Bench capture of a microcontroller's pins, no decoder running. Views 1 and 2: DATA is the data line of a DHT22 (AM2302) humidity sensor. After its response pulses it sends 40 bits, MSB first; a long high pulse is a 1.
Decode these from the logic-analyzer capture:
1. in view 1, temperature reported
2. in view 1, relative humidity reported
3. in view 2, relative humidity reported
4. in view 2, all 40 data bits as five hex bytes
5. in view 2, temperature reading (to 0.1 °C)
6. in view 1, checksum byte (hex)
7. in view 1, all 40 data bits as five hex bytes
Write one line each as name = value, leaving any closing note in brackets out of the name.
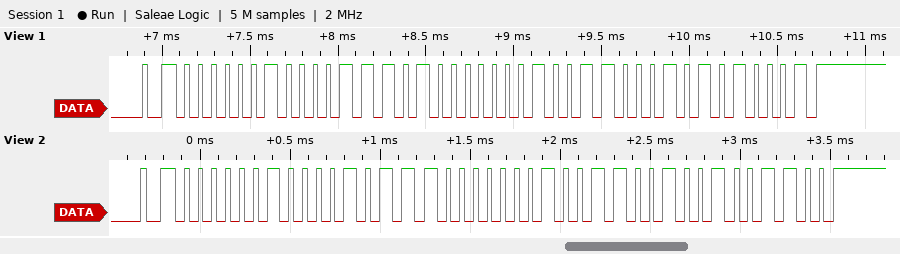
in view 1, temperature reported = 30.5 °C
in view 1, relative humidity reported = 54.1 %
in view 2, relative humidity reported = 53.5 %
in view 2, all 40 data bits as five hex bytes = 02 17 01 32 4C
in view 2, temperature reading = 30.6 °C
in view 1, checksum byte = 0x51
in view 1, all 40 data bits as five hex bytes = 02 1D 01 31 51
